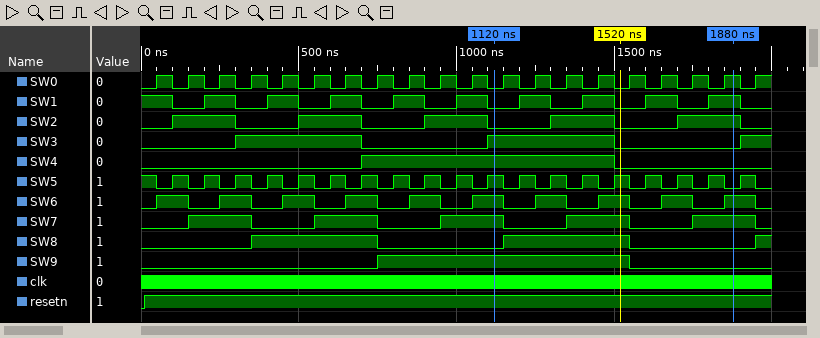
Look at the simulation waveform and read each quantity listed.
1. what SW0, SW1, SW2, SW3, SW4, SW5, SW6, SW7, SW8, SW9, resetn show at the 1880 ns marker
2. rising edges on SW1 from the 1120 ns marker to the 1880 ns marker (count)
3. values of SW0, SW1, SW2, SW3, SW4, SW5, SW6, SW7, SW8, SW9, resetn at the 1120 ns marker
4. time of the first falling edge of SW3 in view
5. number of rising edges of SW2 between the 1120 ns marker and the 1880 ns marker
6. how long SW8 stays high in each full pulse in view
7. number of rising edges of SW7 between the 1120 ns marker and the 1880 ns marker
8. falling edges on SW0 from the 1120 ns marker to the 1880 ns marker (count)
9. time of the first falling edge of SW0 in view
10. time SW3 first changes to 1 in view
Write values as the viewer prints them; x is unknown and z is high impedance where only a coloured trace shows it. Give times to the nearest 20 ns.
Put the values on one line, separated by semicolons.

SW0=1, SW1=1, SW2=1, SW3=0, SW4=0, SW5=0, SW6=1, SW7=1, SW8=0, SW9=0, resetn=1; 4; SW0=0, SW1=0, SW2=0, SW3=1, SW4=1, SW5=1, SW6=1, SW7=1, SW8=0, SW9=1, resetn=1; 700 ns; 2; 400 ns, 400 ns; 2; 7; 100 ns; 300 ns
